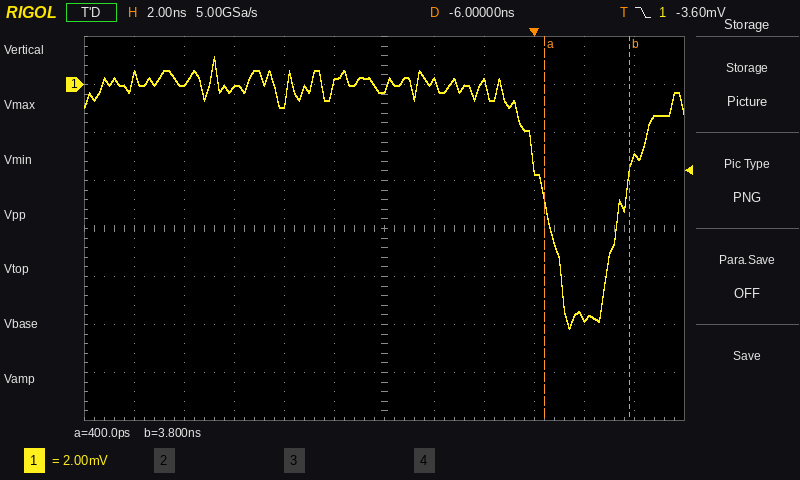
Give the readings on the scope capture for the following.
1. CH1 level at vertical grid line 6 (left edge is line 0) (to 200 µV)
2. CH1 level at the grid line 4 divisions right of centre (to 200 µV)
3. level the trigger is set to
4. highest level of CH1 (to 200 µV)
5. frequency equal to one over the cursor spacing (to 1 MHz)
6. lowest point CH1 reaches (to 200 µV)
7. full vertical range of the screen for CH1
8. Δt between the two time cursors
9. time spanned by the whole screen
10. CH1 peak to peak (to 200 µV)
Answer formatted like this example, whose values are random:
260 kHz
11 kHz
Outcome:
-200 µV
-9.8 mV
-3.60 mV
1.2 mV
294 MHz
-10.2 mV
16 mV
3.4 ns
24 ns
11.4 mV
